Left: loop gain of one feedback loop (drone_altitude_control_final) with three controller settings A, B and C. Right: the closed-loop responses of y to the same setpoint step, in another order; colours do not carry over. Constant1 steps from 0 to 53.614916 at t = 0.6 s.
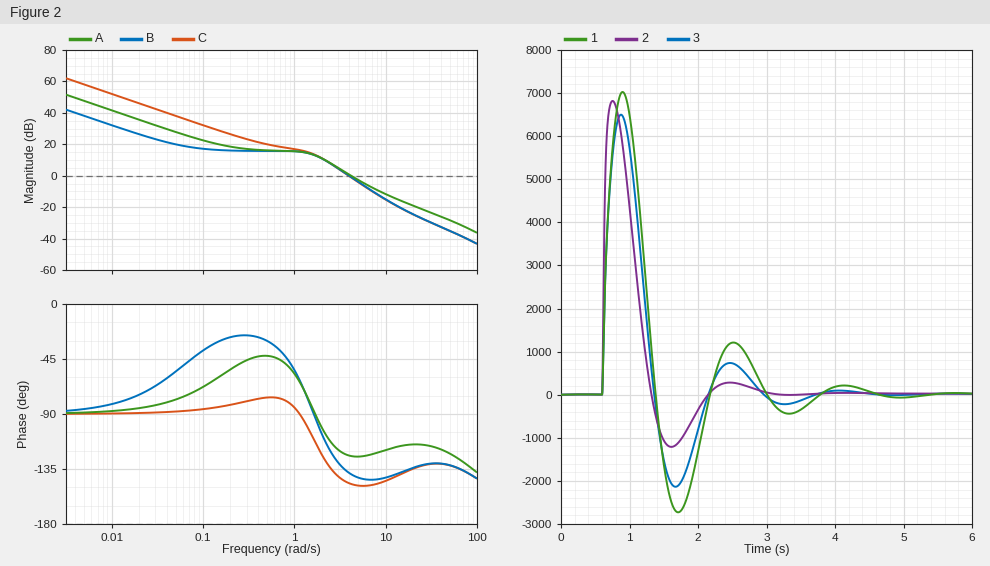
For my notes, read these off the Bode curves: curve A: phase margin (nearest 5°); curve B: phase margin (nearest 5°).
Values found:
55°
40°
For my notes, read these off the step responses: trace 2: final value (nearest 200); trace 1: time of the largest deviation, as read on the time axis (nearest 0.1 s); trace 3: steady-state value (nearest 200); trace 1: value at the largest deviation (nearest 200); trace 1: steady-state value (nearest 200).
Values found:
0
0.9 s
0
7000
0
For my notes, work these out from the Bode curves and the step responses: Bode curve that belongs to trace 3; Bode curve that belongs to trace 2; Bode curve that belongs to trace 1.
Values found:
B
A
C
